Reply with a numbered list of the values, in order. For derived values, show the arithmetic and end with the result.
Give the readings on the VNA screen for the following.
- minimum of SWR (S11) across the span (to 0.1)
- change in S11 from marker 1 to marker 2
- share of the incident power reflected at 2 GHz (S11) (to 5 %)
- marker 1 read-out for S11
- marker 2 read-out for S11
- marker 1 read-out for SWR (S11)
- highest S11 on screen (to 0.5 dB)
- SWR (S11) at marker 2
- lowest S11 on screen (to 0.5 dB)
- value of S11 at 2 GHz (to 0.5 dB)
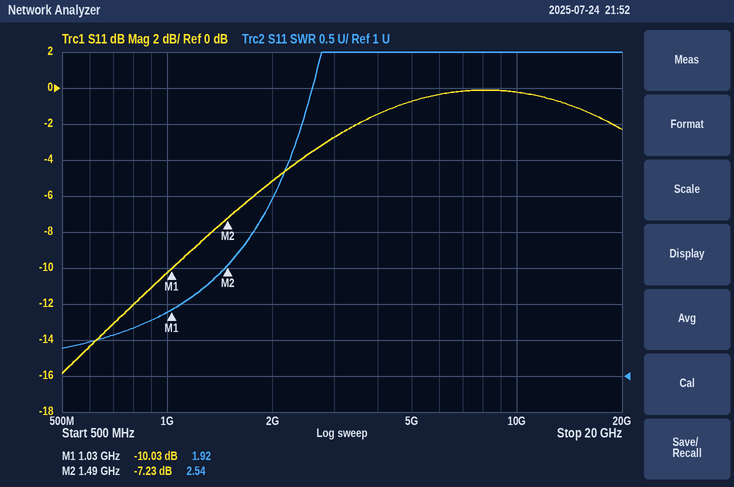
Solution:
1. 1.4
2. -7.23 − (-10.03) = 2.80 dB
3. 10^(-5/10) ≈ 31.6 %, so 30 % to the nearest 5 %
4. -10.03 dB
5. -7.23 dB
6. 1.92
7. 0.0 dB
8. 2.54
9. -16.0 dB
10. -5.0 dB
